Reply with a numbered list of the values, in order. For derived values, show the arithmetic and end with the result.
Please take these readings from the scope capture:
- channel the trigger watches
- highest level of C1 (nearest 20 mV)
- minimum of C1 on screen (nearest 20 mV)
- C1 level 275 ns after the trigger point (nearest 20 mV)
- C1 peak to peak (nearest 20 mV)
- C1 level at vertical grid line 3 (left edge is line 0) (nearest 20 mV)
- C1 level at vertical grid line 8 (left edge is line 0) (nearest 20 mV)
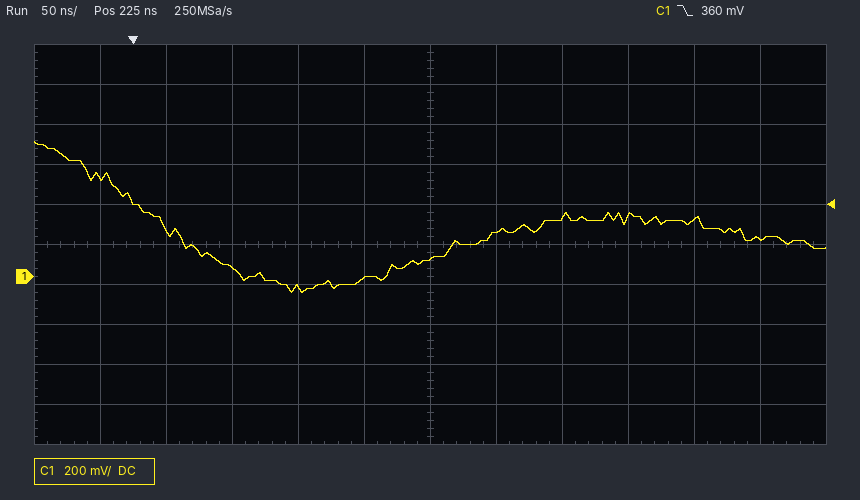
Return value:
1. C1
2. 680 mV
3. -80 mV
4. 220 mV
5. 680 mV − (-80 mV) = 760 mV
6. 40 mV
7. 300 mV
